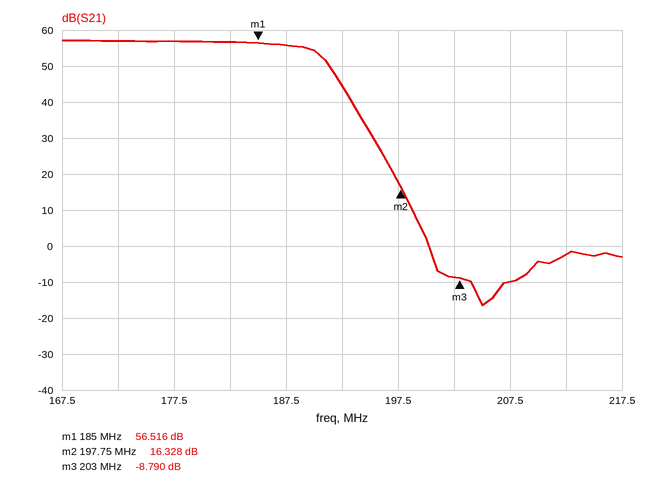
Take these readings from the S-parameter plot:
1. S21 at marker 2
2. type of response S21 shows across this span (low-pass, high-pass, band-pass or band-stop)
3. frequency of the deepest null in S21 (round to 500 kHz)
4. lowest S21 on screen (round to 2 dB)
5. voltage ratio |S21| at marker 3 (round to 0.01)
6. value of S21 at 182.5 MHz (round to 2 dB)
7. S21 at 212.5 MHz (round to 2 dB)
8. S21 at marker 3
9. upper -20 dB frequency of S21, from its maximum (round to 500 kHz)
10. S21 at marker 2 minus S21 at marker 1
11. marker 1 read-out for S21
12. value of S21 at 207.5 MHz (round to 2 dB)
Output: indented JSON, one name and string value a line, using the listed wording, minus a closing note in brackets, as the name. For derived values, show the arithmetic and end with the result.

{
  "S21 at marker 2": "16.328 dB",
  "type of response S21 shows across this span": "low-pass",
  "frequency of the deepest null in S21": "205.0 MHz",
  "lowest S21 on screen": "-16 dB",
  "voltage ratio |S21| at marker 3": "10^(-8.79/20) ≈ 0.36",
  "value of S21 at 182.5 MHz": "56 dB",
  "S21 at 212.5 MHz": "-2 dB",
  "S21 at marker 3": "-8.790 dB",
  "upper -20 dB frequency of S21, from its maximum": "194.0 MHz",
  "S21 at marker 2 minus S21 at marker 1": "16.328 − (56.516) = -40.188 dB",
  "marker 1 read-out for S21": "56.516 dB",
  "value of S21 at 207.5 MHz": "-10 dB"
}
